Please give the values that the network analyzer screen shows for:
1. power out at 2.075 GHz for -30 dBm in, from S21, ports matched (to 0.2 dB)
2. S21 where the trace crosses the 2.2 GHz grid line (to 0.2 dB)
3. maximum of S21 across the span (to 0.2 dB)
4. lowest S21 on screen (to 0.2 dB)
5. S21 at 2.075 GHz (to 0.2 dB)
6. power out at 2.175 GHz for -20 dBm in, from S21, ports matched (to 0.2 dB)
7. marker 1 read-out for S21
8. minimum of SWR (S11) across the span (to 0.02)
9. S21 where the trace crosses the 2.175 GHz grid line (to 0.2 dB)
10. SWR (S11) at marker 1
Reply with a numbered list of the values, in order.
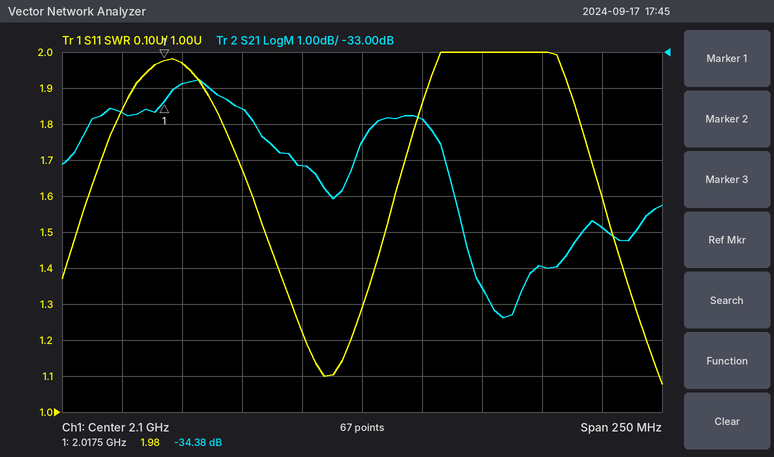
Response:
1. -66.2 dBm
2. -37.8 dB
3. -33.8 dB
4. -40.4 dB
5. -36.2 dB
6. -59.0 dBm
7. -34.38 dB
8. 1.08
9. -39.0 dB
10. 1.98
